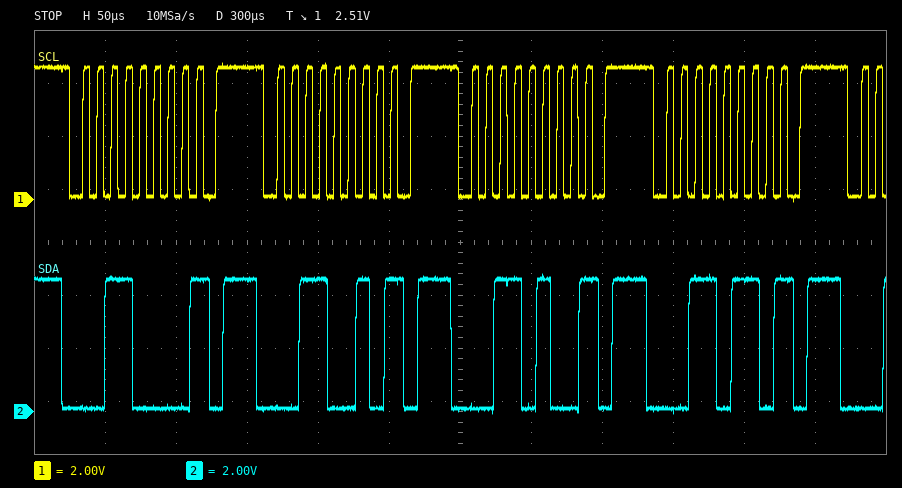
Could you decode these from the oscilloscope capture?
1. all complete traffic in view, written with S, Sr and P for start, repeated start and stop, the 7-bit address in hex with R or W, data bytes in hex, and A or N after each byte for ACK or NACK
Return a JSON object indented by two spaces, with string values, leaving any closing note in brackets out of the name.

{
  "all complete traffic in view, written with S, Sr and P for start, repeated start and stop, the 7-bit address in hex with R or W, data bytes in hex, and A or N after each byte for ACK or NACK": "S 18W N P S 19W N P S 1AW N P S 1BW N P"
}
